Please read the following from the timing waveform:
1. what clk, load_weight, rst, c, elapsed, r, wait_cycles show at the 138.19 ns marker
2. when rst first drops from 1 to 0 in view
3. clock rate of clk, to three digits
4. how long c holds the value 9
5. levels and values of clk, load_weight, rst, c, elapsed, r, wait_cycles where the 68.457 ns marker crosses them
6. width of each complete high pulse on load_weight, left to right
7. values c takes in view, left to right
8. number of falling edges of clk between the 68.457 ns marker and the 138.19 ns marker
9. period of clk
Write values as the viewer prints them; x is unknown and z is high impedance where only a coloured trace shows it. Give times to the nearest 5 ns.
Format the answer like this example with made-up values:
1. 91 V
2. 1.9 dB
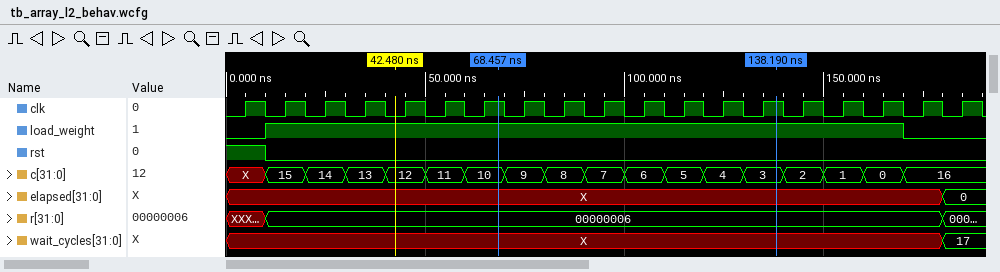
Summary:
1. clk=1, load_weight=1, rst=0, c=3, elapsed=X, r=00000006, wait_cycles=X
2. 10 ns
3. 100 MHz
4. 10 ns
5. clk=1, load_weight=1, rst=0, c=10, elapsed=X, r=00000006, wait_cycles=X
6. 160 ns
7. X, 15, 14, 13, 12, 11, 10, 9, 8, 7, 6, 5, 4, 3, 2, 1, 0, 16
8. 7
9. 10 ns
